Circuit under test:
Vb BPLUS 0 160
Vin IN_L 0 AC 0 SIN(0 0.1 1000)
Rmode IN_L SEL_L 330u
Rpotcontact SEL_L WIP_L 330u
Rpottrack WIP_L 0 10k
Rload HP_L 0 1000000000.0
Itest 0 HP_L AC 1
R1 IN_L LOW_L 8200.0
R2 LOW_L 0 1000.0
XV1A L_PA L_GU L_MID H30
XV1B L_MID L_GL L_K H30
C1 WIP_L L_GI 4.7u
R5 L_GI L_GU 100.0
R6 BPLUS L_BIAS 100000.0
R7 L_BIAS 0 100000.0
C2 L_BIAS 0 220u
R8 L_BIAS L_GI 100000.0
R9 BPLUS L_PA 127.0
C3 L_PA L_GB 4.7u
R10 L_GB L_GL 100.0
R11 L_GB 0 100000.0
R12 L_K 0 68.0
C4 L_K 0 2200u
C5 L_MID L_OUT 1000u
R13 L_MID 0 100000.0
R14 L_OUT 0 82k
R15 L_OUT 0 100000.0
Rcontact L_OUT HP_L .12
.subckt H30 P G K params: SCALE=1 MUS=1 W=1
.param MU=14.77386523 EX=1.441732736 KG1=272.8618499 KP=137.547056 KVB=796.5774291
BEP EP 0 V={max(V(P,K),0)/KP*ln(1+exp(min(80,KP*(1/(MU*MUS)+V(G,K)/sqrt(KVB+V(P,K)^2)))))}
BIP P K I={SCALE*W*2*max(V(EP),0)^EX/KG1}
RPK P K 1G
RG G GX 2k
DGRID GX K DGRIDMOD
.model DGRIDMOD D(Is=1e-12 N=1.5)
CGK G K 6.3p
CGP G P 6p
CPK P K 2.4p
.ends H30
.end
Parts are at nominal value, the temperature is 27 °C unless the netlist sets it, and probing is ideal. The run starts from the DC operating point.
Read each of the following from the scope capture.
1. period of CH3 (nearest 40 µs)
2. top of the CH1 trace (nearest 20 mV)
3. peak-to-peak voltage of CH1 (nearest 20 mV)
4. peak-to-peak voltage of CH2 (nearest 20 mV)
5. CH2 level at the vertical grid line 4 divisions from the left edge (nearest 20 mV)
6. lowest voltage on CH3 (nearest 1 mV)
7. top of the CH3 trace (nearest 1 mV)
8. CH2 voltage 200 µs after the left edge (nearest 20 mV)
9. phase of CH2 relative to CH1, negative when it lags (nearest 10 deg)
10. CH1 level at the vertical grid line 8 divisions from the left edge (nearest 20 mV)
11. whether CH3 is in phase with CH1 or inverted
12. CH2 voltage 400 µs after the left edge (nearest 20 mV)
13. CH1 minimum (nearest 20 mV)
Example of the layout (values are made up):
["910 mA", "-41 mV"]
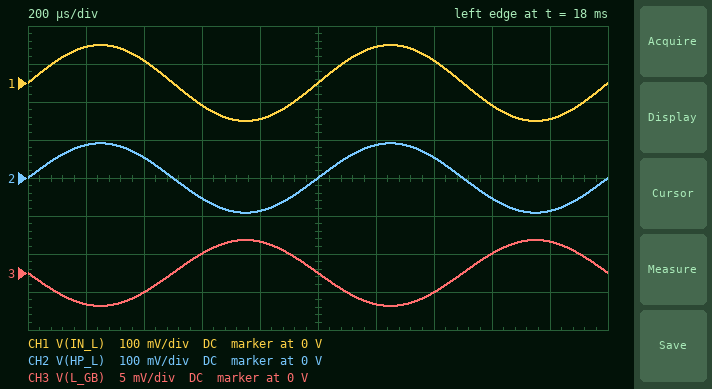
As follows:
["1.00 ms", "100 mV", "200 mV", "180 mV", "-80 mV", "-4 mV", "4 mV", "80 mV", "0 deg", "-60 mV", "inverted", "60 mV", "-100 mV"]
